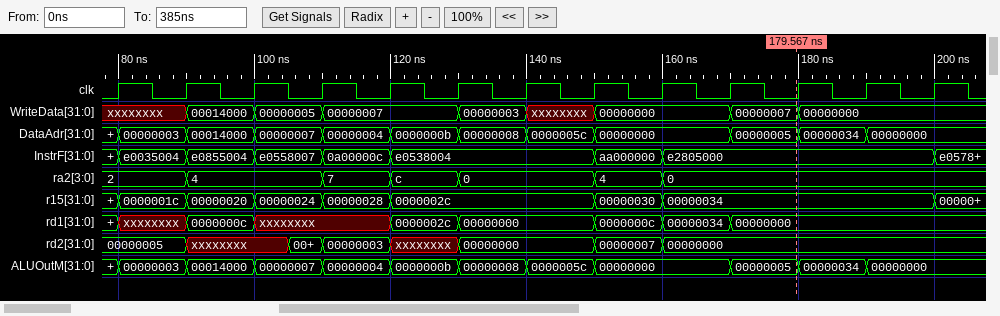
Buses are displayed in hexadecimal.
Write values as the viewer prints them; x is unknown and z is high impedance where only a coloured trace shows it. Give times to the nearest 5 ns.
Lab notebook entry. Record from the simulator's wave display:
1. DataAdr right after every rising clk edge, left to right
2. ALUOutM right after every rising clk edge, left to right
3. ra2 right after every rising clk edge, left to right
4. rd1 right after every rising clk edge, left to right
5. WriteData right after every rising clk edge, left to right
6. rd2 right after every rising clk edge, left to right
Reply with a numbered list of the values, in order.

1. 00000003, 00014000, 00000007, 00000004, 0000000b, 00000008, 0000005c, 00000000, 00000000, 00000005, 00000034, 00000000, 00000000
2. 00000003, 00014000, 00000007, 00000004, 0000000b, 00000008, 0000005c, 00000000, 00000000, 00000005, 00000034, 00000000, 00000000
3. 2, 4, 4, 7, c, 0, 0, 4, 0, 0, 0, 0, 0
4. xxxxxxxx, 0000000c, xxxxxxxx, xxxxxxxx, 0000002c, 00000000, 00000000, 0000000c, 00000034, 00000000, 00000000, 00000000, 00000000
5. xxxxxxxx, 00014000, 00000005, 00000007, 00000007, 00000003, xxxxxxxx, 00000000, 00000000, 00000007, 00000000, 00000000, 00000000
6. 00000005, xxxxxxxx, xxxxxxxx, 00000003, xxxxxxxx, 00000000, 00000000, 00000007, 00000000, 00000000, 00000000, 00000000, 00000000
